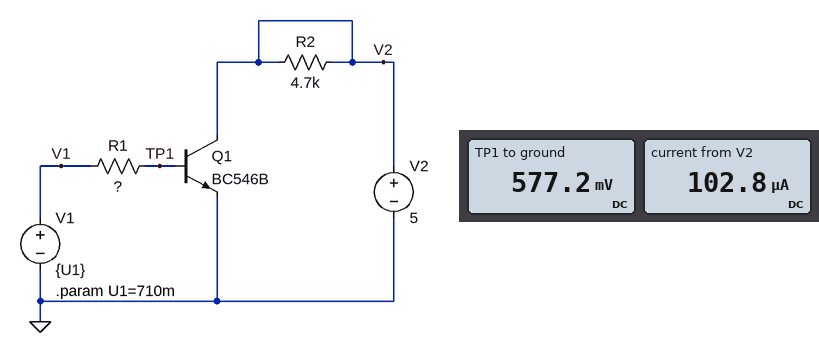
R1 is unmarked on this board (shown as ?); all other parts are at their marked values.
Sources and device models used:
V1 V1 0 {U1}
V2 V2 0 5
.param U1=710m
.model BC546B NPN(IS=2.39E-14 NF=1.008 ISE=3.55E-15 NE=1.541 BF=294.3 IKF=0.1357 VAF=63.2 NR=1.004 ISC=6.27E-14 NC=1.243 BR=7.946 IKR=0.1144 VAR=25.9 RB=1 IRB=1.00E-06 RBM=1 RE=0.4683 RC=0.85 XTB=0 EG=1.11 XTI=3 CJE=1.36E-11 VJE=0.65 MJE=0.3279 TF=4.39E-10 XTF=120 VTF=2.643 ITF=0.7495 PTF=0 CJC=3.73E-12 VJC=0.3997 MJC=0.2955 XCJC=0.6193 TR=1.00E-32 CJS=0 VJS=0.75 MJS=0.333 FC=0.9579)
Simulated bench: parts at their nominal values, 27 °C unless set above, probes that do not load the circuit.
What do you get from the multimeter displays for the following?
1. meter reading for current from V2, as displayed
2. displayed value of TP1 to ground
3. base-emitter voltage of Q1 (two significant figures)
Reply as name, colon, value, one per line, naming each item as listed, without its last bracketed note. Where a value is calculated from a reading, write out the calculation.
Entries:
meter reading for current from V2, as displayed: 102.8 µA
displayed value of TP1 to ground: 577.2 mV
base-emitter voltage of Q1: 577.2 mV = 580 mV
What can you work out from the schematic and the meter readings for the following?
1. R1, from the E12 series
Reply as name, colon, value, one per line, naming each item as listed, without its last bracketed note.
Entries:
R1, from the E12 series: 390 kΩ
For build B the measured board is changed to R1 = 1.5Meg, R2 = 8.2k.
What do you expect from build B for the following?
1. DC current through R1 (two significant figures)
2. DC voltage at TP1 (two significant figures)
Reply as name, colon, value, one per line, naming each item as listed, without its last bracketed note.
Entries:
DC current through R1: 110 nA
DC voltage at TP1: 550 mV
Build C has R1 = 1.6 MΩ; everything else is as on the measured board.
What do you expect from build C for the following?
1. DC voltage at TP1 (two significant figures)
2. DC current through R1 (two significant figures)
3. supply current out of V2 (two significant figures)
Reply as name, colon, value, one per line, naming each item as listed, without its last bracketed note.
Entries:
DC voltage at TP1: 550 mV
DC current through R1: 100 nA
supply current out of V2: 31 µA
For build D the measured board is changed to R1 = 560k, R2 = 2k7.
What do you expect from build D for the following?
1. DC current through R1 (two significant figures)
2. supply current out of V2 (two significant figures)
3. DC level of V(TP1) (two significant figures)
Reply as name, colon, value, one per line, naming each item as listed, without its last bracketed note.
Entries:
DC current through R1: 250 nA
supply current out of V2: 76 µA
DC level of V(TP1): 570 mV
